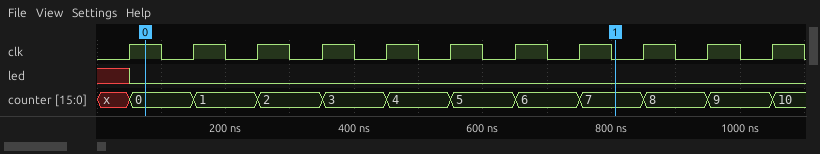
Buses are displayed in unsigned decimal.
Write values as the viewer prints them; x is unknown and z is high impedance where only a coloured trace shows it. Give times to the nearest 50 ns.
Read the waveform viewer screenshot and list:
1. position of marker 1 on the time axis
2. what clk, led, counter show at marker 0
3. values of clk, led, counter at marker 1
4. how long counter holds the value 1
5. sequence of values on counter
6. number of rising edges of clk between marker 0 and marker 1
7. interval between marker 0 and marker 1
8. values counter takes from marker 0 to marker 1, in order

800 ns
clk=1, led=0, counter=0
clk=0, led=0, counter=7
100 ns
x, 0, 1, 2, 3, 4, 5, 6, 7, 8, 9, 10
7
750 ns
0, 1, 2, 3, 4, 5, 6, 7
